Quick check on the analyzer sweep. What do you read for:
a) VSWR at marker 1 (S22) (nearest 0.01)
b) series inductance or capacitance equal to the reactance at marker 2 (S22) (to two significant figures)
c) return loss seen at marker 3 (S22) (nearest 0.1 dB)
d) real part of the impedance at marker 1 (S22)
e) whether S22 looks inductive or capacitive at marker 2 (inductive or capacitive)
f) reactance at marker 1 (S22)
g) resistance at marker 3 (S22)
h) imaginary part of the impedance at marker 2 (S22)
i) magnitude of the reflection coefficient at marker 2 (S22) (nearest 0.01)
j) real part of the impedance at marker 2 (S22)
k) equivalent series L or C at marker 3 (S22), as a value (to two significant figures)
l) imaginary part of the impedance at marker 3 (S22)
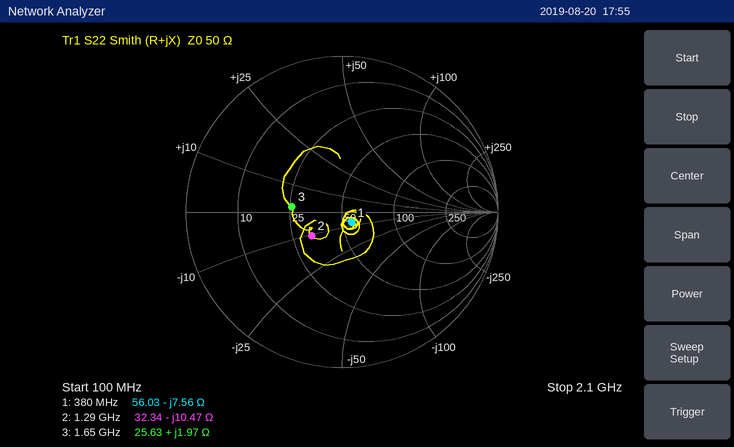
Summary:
1.20
12 pF
9.8 dB
56.03 Ω
capacitive
-7.56 Ω
25.63 Ω
-10.47 Ω
0.25
32.34 Ω
190 pH
+1.97 Ω
